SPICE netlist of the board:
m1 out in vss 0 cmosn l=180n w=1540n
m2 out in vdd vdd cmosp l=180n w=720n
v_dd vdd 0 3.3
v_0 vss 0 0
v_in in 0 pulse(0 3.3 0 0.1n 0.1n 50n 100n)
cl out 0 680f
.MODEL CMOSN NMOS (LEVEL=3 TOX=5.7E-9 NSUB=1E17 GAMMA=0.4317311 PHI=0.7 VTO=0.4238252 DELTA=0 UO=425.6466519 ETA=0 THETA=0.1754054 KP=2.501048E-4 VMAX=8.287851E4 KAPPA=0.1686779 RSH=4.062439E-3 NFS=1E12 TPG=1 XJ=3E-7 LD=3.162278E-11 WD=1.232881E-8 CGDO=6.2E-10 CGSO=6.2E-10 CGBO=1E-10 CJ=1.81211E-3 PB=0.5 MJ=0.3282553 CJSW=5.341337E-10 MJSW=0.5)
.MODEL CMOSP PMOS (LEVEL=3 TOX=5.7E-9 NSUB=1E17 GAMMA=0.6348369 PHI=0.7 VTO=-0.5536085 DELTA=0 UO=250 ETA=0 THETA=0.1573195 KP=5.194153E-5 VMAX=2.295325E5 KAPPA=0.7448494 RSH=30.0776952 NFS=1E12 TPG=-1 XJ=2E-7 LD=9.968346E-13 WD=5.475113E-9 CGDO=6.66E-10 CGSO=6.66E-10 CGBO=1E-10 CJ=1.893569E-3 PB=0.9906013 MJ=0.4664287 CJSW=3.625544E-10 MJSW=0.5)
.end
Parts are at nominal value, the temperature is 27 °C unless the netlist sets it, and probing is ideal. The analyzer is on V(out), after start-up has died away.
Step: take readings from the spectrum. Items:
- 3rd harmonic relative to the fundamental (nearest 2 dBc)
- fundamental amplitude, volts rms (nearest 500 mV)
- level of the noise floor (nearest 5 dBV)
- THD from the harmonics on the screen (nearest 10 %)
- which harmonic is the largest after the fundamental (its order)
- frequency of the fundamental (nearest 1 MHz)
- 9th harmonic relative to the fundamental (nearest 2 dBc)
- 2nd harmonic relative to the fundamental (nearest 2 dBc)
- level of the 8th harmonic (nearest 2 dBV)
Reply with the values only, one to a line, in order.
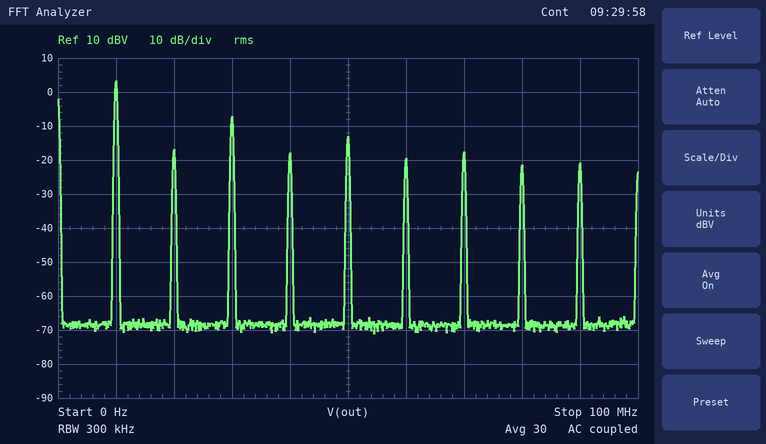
-10 dBc
1.5 V
-70 dBV
40 %
3
10 MHz
-24 dBc
-20 dBc
-22 dBV
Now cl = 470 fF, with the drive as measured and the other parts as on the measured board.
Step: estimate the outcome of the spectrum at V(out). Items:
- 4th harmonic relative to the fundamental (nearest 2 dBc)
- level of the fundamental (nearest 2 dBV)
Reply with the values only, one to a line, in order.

-24 dBc
4 dBV
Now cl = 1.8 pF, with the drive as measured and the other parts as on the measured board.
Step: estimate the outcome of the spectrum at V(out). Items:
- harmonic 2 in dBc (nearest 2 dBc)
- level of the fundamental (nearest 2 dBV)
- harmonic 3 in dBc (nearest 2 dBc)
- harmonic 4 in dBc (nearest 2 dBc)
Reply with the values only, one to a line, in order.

-14 dBc
2 dBV
-14 dBc
-18 dBc
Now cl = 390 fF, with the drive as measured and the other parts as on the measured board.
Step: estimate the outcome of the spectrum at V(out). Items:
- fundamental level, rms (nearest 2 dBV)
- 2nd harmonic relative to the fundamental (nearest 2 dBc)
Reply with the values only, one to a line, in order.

4 dBV
-24 dBc
